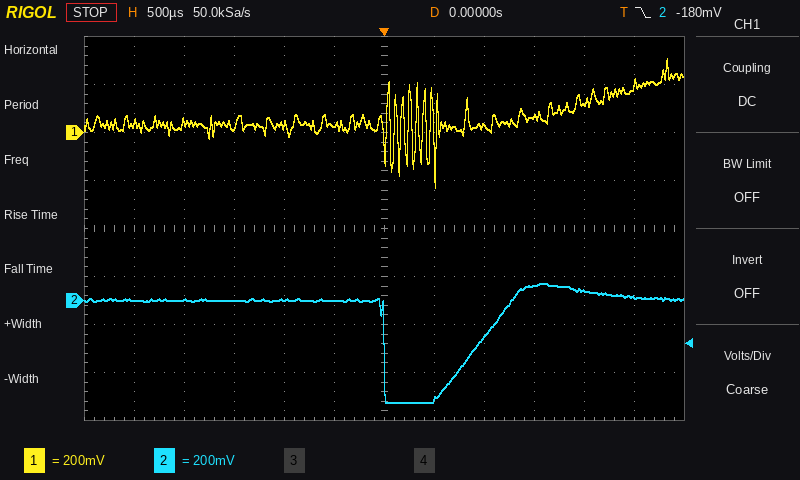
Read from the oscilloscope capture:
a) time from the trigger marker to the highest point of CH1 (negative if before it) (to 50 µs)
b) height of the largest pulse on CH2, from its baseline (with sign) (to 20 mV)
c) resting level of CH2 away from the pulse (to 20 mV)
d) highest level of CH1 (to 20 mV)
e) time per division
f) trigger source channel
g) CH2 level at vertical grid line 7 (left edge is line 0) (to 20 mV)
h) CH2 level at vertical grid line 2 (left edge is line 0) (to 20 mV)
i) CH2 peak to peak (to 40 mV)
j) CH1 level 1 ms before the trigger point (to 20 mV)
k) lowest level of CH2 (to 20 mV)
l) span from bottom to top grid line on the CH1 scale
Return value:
+2.85 ms
-420 mV
0 mV
300 mV
500 µs
CH2
-420 mV
0 mV
480 mV
40 mV
-420 mV
1.6 V
